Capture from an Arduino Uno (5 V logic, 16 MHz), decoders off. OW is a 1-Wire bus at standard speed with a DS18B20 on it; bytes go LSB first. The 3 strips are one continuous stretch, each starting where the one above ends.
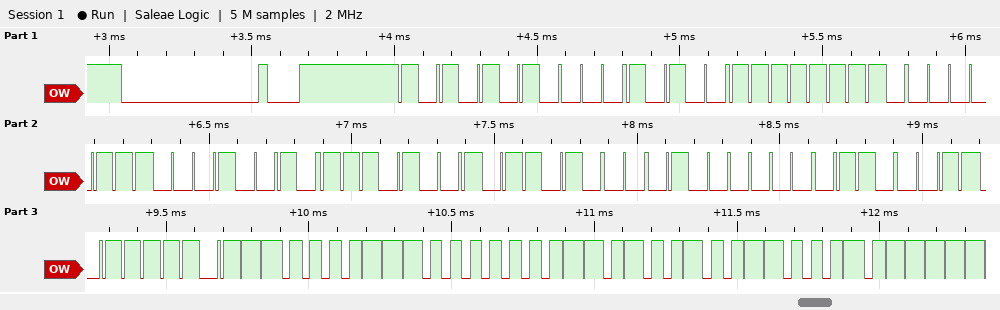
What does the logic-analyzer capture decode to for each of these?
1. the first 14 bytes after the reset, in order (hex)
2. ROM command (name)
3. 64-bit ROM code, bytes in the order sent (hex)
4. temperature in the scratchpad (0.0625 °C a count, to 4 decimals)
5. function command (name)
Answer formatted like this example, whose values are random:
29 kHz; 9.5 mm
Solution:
55 28 FF E0 48 97 16 02 C6 BE C3 01 4B 46; Match ROM; 28 FF E0 48 97 16 02 C6; 28.1875 °C; Read Scratchpad
